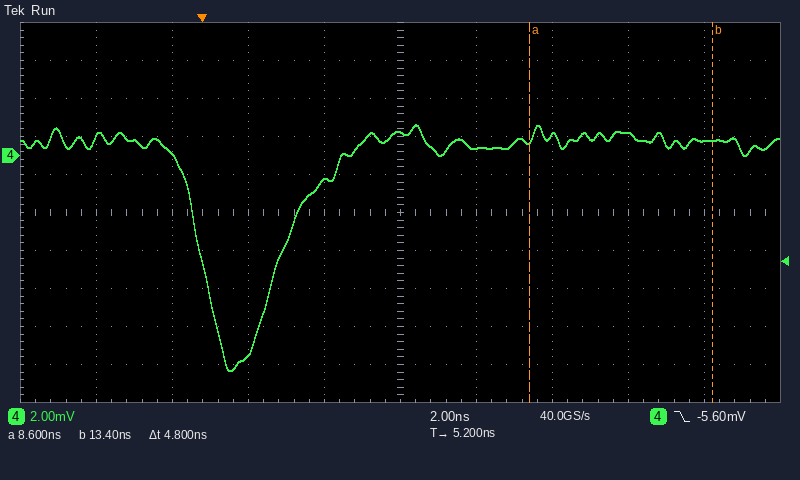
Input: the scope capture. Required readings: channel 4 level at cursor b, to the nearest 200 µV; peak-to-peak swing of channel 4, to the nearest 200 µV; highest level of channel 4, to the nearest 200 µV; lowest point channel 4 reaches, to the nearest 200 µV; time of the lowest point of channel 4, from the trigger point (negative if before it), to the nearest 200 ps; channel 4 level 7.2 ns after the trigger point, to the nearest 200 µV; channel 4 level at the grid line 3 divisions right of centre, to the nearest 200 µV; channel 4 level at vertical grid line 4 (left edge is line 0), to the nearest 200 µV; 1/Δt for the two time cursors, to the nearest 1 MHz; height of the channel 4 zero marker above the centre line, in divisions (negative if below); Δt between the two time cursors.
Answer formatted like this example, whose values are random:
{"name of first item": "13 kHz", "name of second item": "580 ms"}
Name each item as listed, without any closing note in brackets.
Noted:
{"channel 4 level at cursor b, to the nearest 200 µV": "800 µV", "peak-to-peak swing of channel 4, to the nearest 200 µV": "13.0 mV", "highest level of channel 4, to the nearest 200 µV": "1.6 mV", "lowest point channel 4 reaches, to the nearest 200 µV": "-11.4 mV", "time of the lowest point of channel 4, from the trigger point (negative if before it), to the nearest 200 ps": "+800 ps", "channel 4 level 7.2 ns after the trigger point, to the nearest 200 µV": "400 µV", "channel 4 level at the grid line 3 divisions right of centre, to the nearest 200 µV": "1.2 mV", "channel 4 level at vertical grid line 4 (left edge is line 0), to the nearest 200 µV": "-1.4 mV", "1/Δt for the two time cursors, to the nearest 1 MHz": "208 MHz", "height of the channel 4 zero marker above the centre line, in divisions": "+1.5 div", "Δt between the two time cursors": "4.8 ns"}
